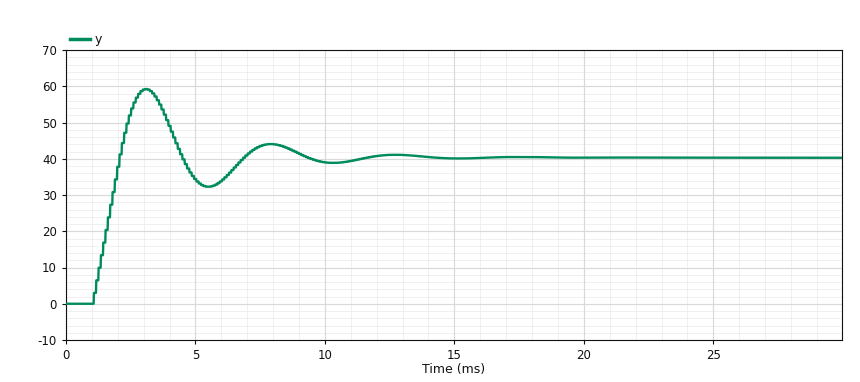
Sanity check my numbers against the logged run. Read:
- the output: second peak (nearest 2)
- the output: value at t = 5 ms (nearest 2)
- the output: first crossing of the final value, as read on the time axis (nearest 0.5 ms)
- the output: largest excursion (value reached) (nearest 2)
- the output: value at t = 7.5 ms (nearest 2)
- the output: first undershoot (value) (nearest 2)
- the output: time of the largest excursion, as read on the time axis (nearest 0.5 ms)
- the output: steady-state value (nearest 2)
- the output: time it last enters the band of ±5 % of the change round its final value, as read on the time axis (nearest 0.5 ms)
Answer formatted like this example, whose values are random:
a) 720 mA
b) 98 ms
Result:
a) 44
b) 34
c) 2.0 ms
d) 60
e) 44
f) 32
g) 3.0 ms
h) 40
i) 9.0 ms
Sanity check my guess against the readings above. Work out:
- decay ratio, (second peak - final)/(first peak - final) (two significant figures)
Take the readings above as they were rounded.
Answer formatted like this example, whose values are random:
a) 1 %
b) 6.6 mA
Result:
a) 0.20
